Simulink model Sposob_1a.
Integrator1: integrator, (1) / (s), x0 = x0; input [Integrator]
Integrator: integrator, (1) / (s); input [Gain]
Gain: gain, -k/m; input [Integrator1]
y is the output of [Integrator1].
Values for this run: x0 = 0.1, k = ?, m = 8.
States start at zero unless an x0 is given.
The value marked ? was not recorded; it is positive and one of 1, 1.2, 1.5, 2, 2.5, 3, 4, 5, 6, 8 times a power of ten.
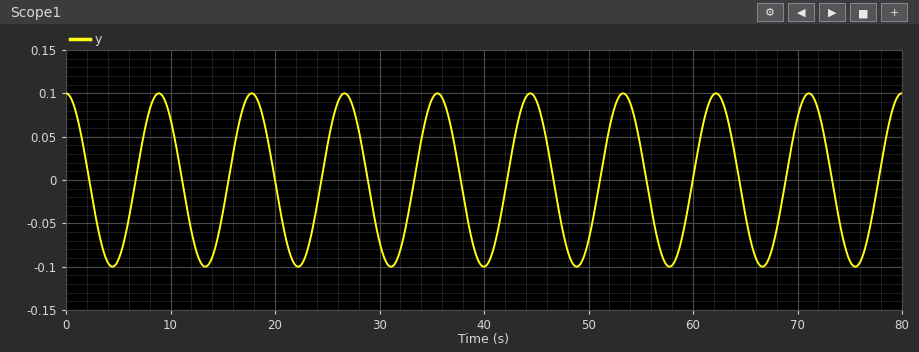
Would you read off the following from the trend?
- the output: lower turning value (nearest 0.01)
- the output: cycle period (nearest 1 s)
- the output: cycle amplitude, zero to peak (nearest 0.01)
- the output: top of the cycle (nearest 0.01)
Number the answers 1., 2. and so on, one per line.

1. -0.10
2. 9 s
3. 0.10
4. 0.10
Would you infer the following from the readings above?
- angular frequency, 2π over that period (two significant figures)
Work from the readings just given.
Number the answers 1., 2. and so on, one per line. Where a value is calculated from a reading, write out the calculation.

1. 2π / 9 = 0.70 rad/s
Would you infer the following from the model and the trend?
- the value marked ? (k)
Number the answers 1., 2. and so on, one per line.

1. 4
